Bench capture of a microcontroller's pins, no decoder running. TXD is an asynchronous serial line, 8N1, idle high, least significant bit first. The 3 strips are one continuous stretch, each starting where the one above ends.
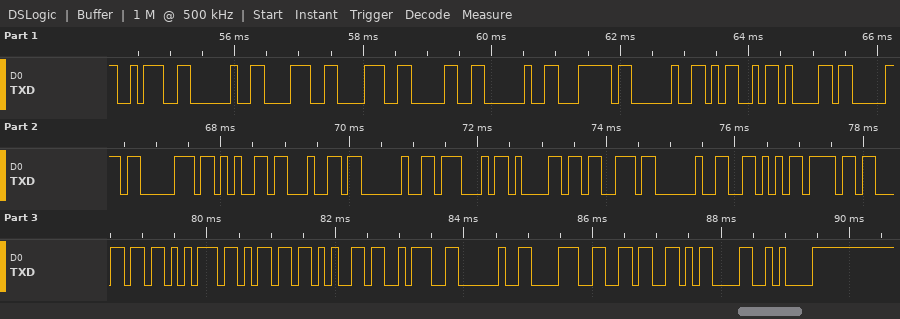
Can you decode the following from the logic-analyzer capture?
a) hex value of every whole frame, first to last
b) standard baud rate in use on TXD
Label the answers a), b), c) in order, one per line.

a) 3A 20 38 38 30 20 7C 20 4D 61 70 70 65 64 20 47 61 73 20 56 6F 6C 75 6D 65 3A 20 38 36 0D 0A
b) 9600 baud
